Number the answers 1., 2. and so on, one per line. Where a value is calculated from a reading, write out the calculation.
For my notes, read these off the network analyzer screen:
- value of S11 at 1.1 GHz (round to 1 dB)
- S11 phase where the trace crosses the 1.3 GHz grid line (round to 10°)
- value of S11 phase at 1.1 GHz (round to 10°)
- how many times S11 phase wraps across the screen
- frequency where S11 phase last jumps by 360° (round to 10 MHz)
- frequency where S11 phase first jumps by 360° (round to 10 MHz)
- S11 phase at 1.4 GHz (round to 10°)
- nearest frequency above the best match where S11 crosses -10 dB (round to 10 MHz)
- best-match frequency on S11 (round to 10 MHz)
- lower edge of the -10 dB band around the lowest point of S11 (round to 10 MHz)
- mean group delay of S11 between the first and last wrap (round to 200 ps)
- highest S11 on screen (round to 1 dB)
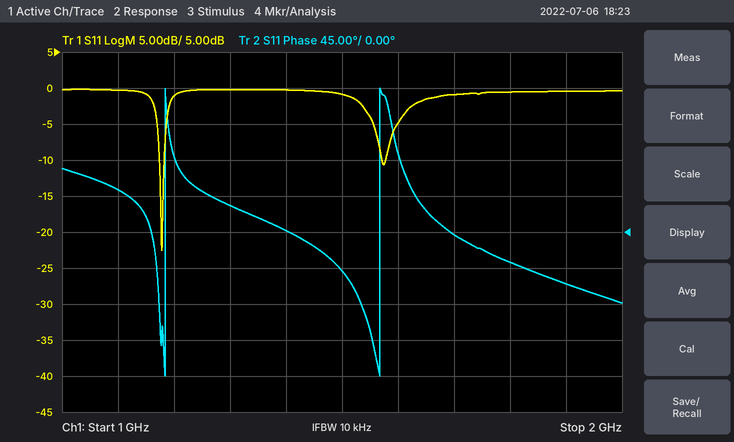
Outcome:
1. 0 dB
2. 30°
3. 50°
4. 2
5. 1.57 GHz
6. 1.18 GHz
7. 0°
8. 1.18 GHz
9. 1.18 GHz
10. 1.17 GHz
11. 1 cycle / (1.57 GHz − 1.18 GHz) ≈ 2.6 ns
12. 0 dB
